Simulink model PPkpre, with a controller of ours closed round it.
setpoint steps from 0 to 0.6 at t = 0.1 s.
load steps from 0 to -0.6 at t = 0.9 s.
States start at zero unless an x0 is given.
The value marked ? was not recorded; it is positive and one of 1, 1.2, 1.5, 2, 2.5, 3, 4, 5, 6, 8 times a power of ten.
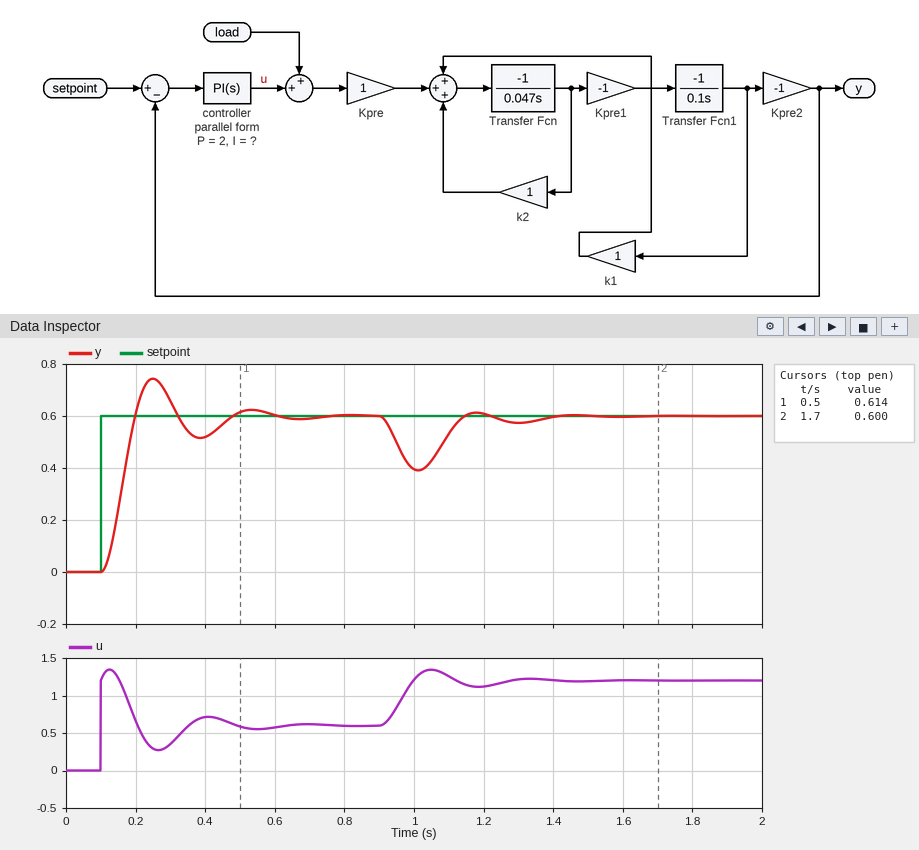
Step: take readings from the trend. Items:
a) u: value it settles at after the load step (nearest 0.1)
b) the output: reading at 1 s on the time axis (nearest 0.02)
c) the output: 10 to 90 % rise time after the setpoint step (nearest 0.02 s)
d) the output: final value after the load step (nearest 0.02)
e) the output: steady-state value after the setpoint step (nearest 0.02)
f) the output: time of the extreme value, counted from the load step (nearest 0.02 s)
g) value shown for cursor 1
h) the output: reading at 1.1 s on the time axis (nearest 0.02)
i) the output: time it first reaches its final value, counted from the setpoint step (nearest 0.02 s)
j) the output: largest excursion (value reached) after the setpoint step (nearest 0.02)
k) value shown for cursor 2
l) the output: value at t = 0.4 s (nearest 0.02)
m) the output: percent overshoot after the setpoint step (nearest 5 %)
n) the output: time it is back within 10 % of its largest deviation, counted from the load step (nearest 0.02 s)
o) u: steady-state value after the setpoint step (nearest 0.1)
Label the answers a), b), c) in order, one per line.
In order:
a) 1.2
b) 0.40
c) 0.06 s
d) 0.60
e) 0.60
f) 0.12 s
g) 0.614
h) 0.54
i) 0.10 s
j) 0.74
k) 0.600
l) 0.52
m) 25 %
n) 0.44 s
o) 0.6
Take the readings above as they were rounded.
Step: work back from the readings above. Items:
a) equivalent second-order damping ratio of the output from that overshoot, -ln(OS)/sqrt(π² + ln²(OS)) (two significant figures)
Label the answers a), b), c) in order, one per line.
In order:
a) 0.40
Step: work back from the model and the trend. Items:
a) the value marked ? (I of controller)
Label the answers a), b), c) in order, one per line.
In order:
a) 20
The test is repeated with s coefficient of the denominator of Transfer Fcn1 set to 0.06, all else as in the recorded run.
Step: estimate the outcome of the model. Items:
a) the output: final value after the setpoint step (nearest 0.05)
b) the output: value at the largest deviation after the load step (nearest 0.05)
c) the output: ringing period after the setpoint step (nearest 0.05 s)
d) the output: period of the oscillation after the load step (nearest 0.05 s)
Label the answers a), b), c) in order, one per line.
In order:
a) 0.60
b) 0.35
c) 0.20 s
d) 0.20 s
